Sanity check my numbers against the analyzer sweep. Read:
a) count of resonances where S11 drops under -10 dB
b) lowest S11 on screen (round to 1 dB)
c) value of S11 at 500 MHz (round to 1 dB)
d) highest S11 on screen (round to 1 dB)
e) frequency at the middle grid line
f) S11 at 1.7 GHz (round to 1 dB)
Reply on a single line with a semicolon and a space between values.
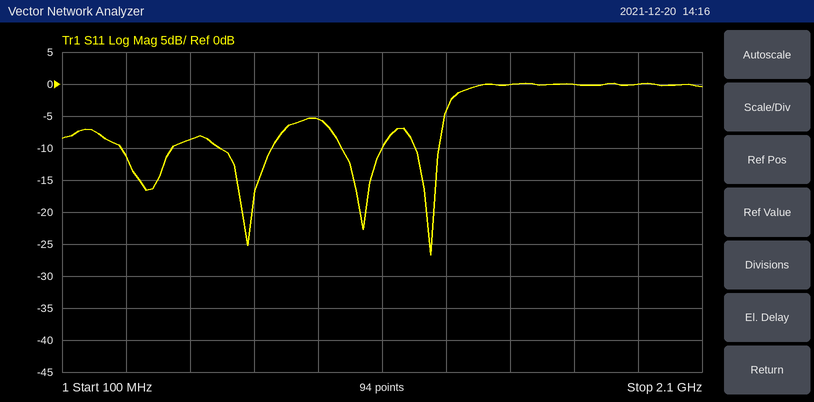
4; -27 dB; -9 dB; 0 dB; 1.1 GHz; 0 dB
